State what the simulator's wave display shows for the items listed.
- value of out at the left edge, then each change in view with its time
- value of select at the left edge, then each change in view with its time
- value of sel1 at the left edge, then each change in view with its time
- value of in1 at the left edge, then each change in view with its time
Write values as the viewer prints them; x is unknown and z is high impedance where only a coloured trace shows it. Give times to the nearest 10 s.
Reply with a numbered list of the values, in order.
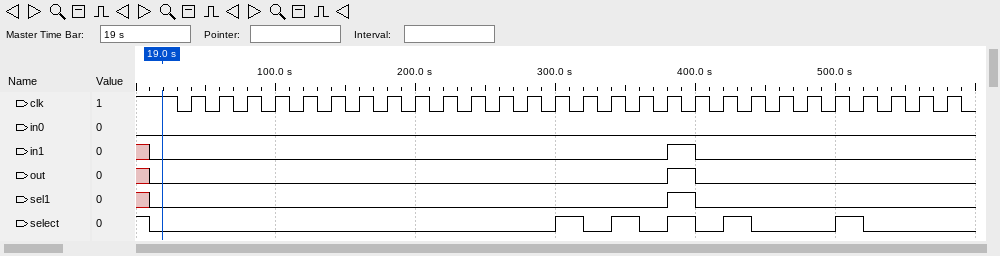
1. x, 0 at 10 s, 1 at 380 s, 0 at 400 s
2. 1, 0 at 10 s, 1 at 300 s, 0 at 320 s, 1 at 340 s, 0 at 360 s, 1 at 380 s, 0 at 400 s, 1 at 420 s, 0 at 440 s, 1 at 500 s, 0 at 520 s
3. x, 0 at 10 s, 1 at 380 s, 0 at 400 s
4. x, 0 at 10 s, 1 at 380 s, 0 at 400 s
